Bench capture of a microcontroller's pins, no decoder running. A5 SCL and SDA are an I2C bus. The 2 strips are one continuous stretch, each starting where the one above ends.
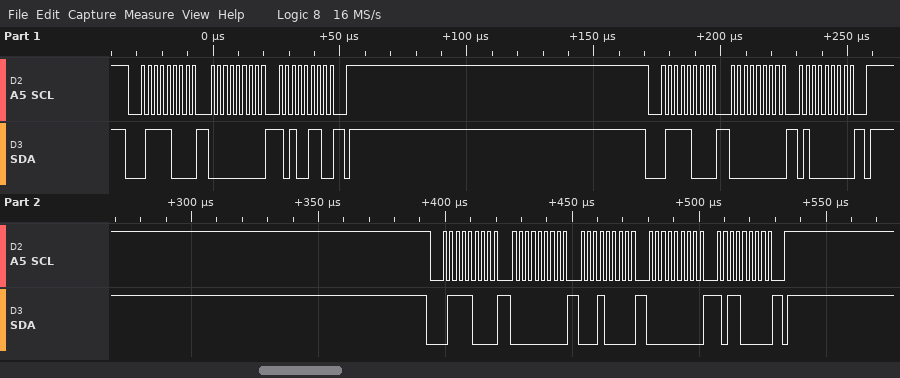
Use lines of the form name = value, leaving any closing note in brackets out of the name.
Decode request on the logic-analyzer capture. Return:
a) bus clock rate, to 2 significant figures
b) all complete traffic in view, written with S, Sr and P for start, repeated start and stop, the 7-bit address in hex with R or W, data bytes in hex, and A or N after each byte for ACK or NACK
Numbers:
bus clock rate, to 2 significant figures = 400 kHz
all complete traffic in view, written with S, Sr and P for start, repeated start and stop, the 7-bit address in hex with R or W, data bytes in hex, and A or N after each byte for ACK or NACK = S 3CW A 00 A A6 A P S 3CW A 00 A 40 A P S 3CW A 00 A 10 A 00 A B0 A P
